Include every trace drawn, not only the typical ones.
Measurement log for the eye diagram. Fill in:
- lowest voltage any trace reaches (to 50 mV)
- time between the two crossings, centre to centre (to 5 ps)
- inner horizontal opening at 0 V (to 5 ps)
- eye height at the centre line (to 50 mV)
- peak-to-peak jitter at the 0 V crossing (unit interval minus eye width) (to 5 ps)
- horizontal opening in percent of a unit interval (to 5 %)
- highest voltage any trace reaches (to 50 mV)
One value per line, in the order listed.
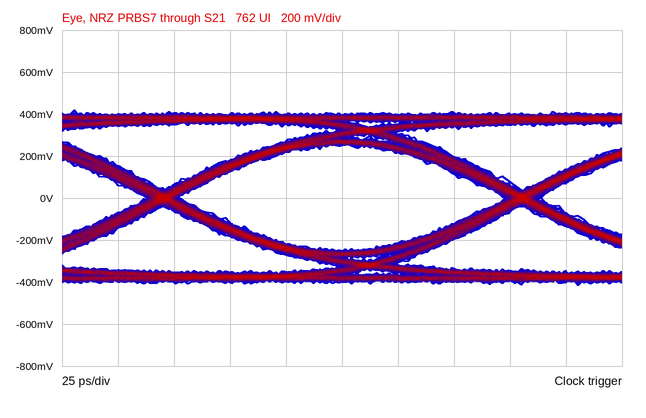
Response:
-400 mV
160 ps
145 ps
500 mV
15 ps
90 %
400 mV
